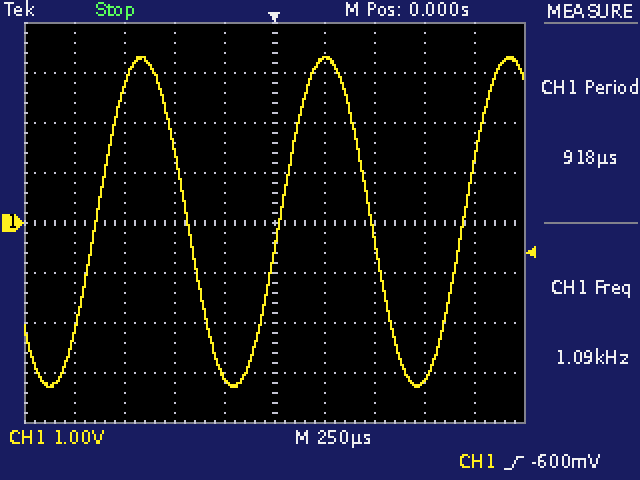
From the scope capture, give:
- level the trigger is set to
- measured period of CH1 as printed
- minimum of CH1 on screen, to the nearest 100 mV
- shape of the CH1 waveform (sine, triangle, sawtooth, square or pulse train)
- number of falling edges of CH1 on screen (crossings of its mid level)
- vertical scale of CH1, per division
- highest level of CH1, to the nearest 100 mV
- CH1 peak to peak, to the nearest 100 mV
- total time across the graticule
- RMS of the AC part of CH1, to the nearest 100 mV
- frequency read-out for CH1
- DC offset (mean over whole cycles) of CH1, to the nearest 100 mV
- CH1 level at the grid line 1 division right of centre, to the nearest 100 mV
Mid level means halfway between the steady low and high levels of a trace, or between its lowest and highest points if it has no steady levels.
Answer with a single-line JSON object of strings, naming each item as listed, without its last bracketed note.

{"level the trigger is set to": "-600 mV", "measured period of CH1 as printed": "918 µs", "minimum of CH1 on screen, to the nearest 100 mV": "-3.3 V", "shape of the CH1 waveform": "sine", "number of falling edges of CH1 on screen": "2", "vertical scale of CH1, per division": "1 V", "highest level of CH1, to the nearest 100 mV": "3.3 V", "CH1 peak to peak, to the nearest 100 mV": "6.6 V", "total time across the graticule": "2.5 ms", "RMS of the AC part of CH1, to the nearest 100 mV": "2.3 V", "frequency read-out for CH1": "1.09 kHz", "DC offset (mean over whole cycles) of CH1, to the nearest 100 mV": "0.0 V", "CH1 level at the grid line 1 division right of centre, to the nearest 100 mV": "3.3 V"}
